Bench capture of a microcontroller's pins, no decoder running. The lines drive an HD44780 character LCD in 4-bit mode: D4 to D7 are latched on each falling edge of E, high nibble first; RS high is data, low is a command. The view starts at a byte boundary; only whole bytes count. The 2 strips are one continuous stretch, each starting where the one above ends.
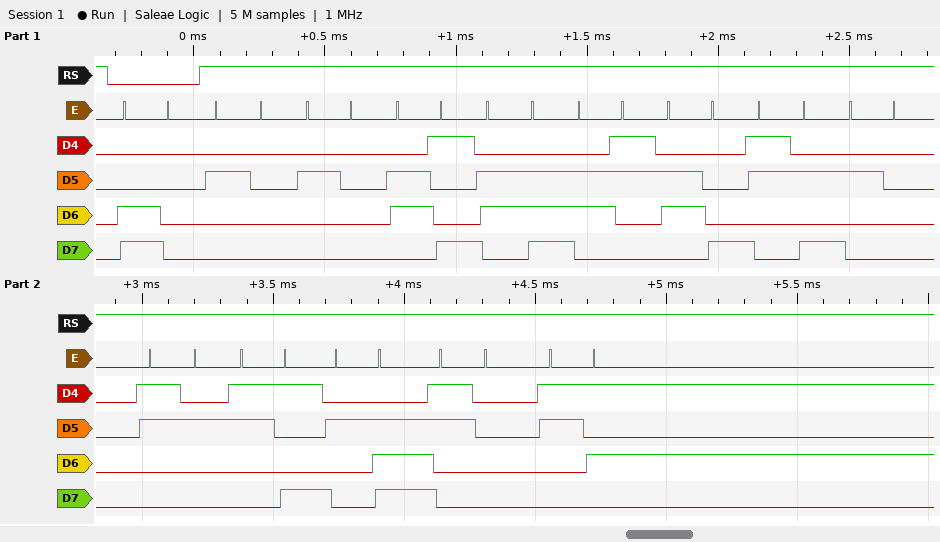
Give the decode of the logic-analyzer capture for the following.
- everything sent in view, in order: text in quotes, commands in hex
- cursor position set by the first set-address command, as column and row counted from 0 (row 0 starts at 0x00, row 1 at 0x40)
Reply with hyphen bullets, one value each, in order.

- 0xC0 "  inch: 29.05"
- column 0, row 1
